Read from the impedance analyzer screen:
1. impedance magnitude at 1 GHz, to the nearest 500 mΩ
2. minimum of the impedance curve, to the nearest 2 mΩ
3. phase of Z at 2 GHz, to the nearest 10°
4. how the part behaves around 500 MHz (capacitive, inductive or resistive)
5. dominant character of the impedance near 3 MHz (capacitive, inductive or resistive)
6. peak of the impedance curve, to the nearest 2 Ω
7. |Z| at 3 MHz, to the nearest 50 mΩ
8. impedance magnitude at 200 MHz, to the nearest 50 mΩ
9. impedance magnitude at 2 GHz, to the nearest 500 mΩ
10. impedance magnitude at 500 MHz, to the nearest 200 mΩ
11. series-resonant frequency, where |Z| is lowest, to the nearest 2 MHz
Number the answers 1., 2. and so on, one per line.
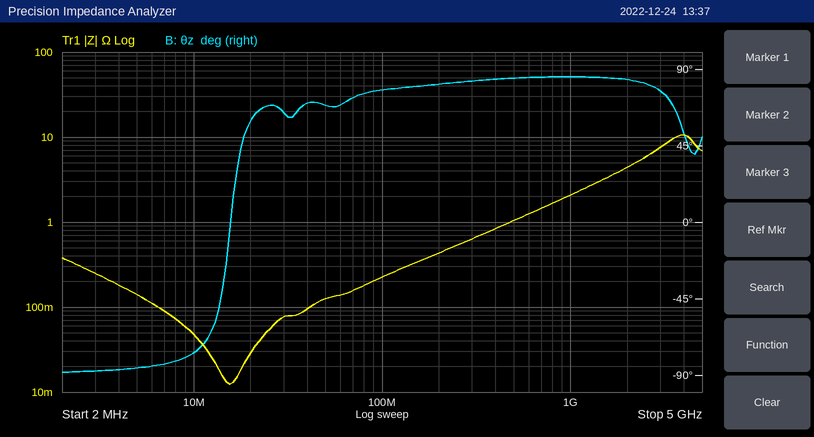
1. 2.0 Ω
2. 12 mΩ
3. 80°
4. inductive
5. capacitive
6. 10 Ω
7. 250 mΩ
8. 450 mΩ
9. 4.5 Ω
10. 1.0 Ω
11. 16 MHz
